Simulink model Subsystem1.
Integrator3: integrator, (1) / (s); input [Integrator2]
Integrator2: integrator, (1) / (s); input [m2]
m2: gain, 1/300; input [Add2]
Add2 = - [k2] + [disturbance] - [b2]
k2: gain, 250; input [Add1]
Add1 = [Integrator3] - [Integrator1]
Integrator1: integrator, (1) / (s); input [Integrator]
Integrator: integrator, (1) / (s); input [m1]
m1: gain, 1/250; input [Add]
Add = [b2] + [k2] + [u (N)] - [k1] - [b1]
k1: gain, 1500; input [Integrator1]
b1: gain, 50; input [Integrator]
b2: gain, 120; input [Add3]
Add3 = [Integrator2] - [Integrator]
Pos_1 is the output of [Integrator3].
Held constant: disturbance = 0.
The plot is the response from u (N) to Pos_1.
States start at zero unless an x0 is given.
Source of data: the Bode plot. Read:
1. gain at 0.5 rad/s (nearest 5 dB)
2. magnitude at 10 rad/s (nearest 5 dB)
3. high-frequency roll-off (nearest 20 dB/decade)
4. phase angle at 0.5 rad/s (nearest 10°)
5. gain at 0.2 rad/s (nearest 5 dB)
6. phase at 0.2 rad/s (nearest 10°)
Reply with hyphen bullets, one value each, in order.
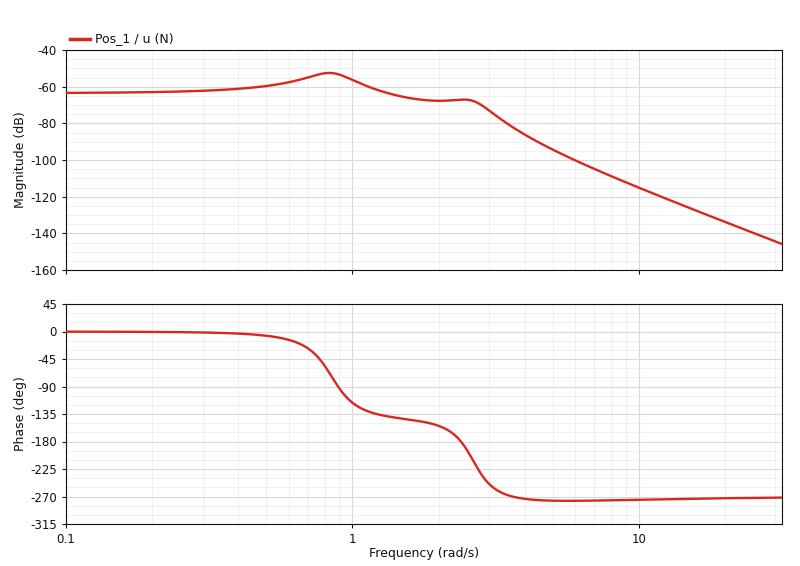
- -60 dB
- -115 dB
- -60 dB/decade
- -10°
- -65 dB
- 0°
